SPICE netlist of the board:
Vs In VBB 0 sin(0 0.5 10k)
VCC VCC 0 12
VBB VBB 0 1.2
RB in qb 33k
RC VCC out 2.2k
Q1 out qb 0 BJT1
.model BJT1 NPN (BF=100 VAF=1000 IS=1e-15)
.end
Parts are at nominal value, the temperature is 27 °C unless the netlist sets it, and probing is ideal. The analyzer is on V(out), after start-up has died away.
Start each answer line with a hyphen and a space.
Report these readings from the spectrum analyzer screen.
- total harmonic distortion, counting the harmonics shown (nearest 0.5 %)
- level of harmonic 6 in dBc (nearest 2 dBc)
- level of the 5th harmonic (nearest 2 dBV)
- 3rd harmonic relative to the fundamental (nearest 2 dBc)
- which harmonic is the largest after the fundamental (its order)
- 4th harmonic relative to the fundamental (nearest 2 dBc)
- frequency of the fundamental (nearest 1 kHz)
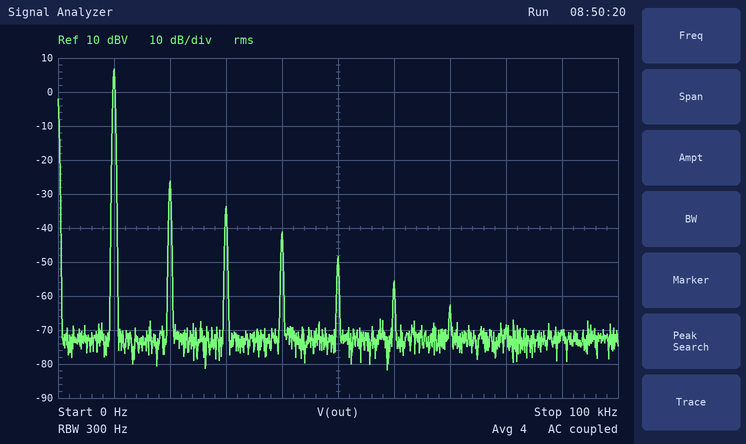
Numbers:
- 2.5 %
- -62 dBc
- -48 dBV
- -40 dBc
- 2
- -48 dBc
- 10 kHz
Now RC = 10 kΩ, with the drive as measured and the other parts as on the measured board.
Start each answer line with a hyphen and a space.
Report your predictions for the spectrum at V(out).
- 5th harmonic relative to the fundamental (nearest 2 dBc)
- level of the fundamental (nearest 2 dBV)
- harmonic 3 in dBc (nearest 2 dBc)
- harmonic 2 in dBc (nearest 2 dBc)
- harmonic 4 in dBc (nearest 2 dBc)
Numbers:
- -24 dBc
- 12 dBV
- -22 dBc
- -6 dBc
- -20 dBc
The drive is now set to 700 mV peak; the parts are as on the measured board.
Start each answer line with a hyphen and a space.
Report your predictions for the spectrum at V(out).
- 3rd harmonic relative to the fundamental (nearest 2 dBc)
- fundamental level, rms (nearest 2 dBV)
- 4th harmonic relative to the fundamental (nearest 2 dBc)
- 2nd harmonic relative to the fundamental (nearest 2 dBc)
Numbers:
- -26 dBc
- 10 dBV
- -32 dBc
- -22 dBc
